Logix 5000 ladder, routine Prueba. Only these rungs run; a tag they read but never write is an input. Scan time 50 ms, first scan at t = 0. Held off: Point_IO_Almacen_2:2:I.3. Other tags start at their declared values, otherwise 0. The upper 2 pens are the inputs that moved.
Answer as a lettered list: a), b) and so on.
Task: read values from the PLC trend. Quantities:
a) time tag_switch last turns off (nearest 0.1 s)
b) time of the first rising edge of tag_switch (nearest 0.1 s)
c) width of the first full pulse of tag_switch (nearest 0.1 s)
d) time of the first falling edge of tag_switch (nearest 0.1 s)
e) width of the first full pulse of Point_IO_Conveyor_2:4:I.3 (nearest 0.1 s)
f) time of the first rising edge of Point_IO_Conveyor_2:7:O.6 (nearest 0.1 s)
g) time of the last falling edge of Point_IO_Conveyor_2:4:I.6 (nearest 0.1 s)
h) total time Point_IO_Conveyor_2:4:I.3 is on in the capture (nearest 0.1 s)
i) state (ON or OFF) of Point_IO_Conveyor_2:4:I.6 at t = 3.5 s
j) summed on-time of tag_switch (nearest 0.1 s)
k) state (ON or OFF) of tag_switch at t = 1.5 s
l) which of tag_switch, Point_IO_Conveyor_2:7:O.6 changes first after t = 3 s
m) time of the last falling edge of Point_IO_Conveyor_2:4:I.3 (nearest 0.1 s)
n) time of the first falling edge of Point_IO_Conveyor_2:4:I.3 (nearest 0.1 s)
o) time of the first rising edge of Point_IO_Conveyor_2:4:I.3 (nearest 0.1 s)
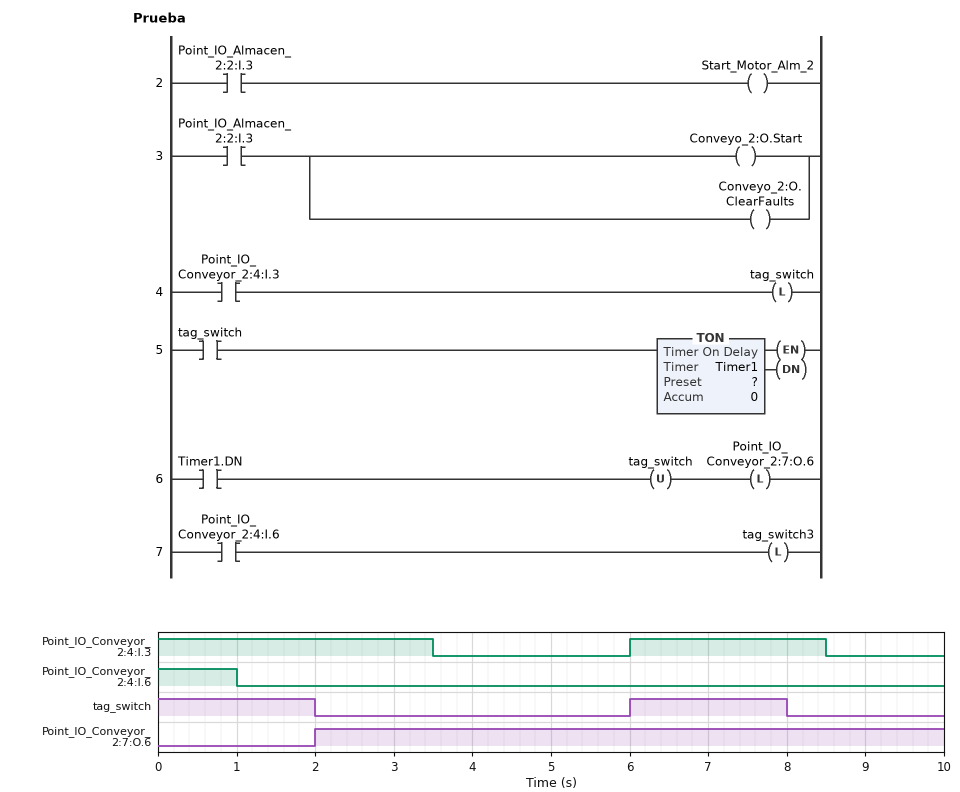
a) 8.0 s
b) 6.0 s
c) 2.0 s
d) 2.0 s
e) 2.5 s
f) 2.0 s
g) 1.0 s
h) 6.0 s
i) OFF
j) 4.0 s
k) ON
l) tag_switch
m) 8.5 s
n) 3.5 s
o) 6.0 s
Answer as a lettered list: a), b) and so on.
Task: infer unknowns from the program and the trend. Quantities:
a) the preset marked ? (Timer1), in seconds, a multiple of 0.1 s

a) 2.0 s
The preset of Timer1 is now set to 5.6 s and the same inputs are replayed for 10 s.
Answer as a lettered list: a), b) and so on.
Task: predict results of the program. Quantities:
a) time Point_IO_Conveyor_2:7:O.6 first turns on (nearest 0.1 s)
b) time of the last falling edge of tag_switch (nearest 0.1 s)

a) 5.6 s
b) 5.6 s
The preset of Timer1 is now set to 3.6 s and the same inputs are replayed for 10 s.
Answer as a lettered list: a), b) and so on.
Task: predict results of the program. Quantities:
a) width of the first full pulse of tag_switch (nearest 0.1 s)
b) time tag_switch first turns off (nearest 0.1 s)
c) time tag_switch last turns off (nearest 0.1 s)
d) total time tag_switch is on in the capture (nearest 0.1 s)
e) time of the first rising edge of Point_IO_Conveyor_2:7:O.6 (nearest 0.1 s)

a) 3.6 s
b) 3.6 s
c) 9.6 s
d) 7.2 s
e) 3.6 s
